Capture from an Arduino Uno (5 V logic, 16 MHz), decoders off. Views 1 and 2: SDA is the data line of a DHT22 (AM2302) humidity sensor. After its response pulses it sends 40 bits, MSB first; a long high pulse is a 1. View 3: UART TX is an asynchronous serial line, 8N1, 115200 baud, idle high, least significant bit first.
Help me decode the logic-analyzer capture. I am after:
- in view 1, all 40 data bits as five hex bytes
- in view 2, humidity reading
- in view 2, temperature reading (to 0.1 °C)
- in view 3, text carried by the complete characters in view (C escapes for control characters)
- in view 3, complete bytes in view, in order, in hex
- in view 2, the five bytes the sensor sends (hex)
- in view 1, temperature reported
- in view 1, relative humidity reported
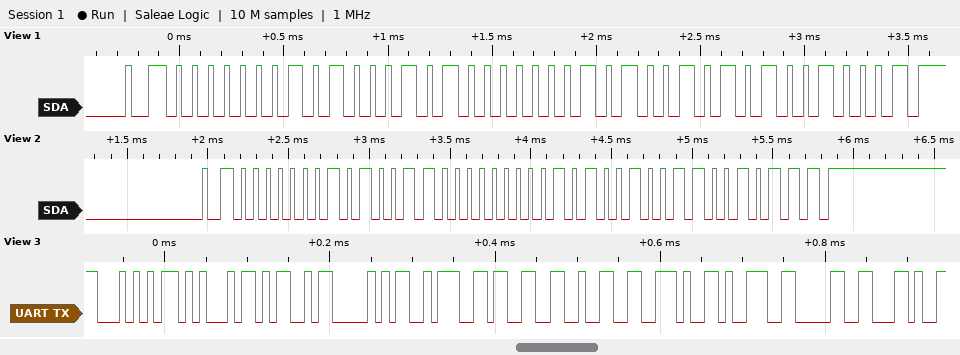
01 45 01 4A 91
33.2 %
32.9 °C
"TEMP:32.90,"
54 45 4D 50 3A 33 32 2E 39 30 2C
01 4C 01 49 97
33.0 °C
32.5 %
